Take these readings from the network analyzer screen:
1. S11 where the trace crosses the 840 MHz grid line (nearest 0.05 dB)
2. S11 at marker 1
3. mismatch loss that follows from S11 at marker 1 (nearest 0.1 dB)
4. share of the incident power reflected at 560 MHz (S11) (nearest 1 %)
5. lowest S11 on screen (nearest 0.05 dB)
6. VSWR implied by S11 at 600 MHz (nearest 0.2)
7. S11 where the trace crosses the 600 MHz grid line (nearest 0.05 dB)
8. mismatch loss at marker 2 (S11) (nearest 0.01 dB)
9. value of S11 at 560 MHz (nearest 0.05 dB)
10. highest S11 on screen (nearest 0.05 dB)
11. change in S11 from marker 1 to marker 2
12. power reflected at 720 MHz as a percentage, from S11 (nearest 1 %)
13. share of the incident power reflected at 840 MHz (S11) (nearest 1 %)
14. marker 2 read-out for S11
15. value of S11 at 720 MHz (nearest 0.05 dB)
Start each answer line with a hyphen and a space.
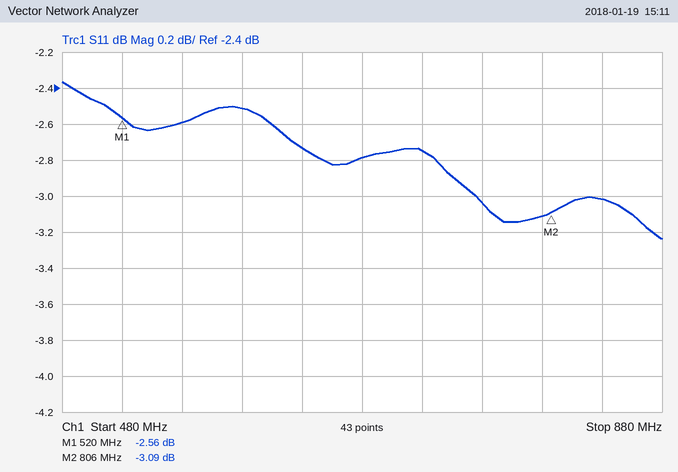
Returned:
- -3.00 dB
- -2.56 dB
- 3.5 dB
- 55 %
- -3.25 dB
- 7.0
- -2.50 dB
- 2.93 dB
- -2.60 dB
- -2.35 dB
- -0.53 dB
- 53 %
- 50 %
- -3.09 dB
- -2.75 dB
